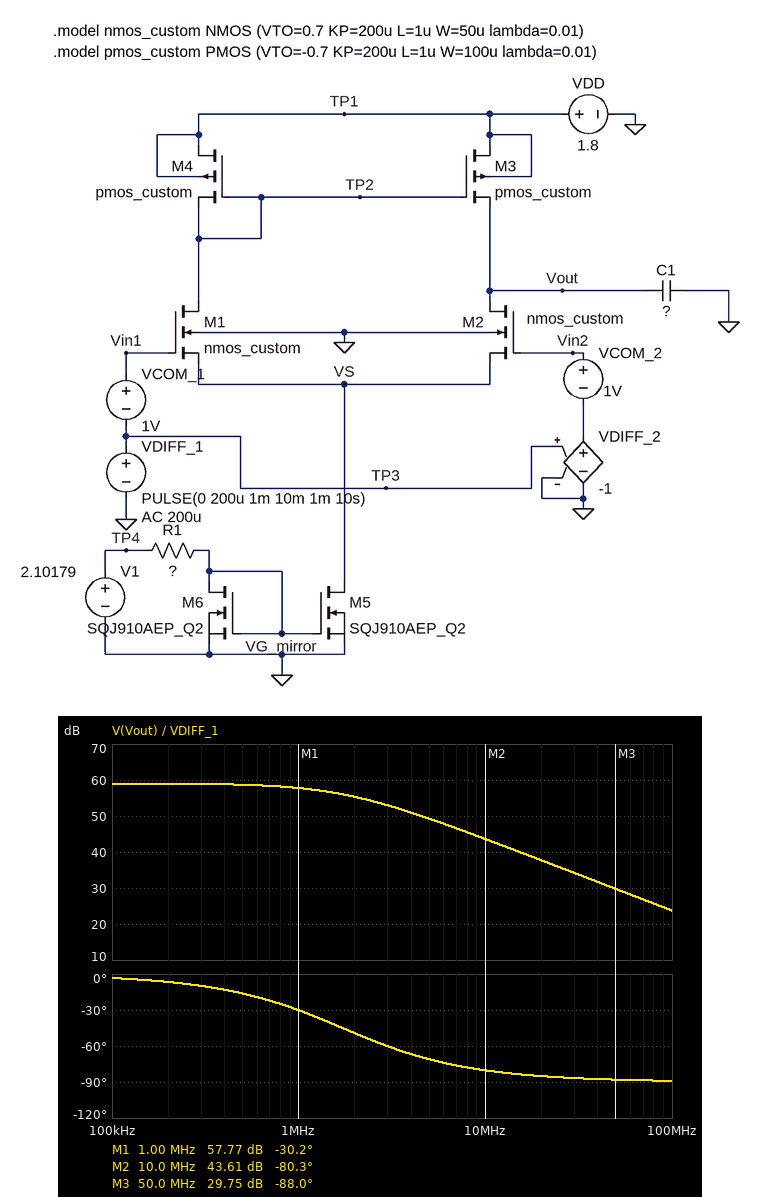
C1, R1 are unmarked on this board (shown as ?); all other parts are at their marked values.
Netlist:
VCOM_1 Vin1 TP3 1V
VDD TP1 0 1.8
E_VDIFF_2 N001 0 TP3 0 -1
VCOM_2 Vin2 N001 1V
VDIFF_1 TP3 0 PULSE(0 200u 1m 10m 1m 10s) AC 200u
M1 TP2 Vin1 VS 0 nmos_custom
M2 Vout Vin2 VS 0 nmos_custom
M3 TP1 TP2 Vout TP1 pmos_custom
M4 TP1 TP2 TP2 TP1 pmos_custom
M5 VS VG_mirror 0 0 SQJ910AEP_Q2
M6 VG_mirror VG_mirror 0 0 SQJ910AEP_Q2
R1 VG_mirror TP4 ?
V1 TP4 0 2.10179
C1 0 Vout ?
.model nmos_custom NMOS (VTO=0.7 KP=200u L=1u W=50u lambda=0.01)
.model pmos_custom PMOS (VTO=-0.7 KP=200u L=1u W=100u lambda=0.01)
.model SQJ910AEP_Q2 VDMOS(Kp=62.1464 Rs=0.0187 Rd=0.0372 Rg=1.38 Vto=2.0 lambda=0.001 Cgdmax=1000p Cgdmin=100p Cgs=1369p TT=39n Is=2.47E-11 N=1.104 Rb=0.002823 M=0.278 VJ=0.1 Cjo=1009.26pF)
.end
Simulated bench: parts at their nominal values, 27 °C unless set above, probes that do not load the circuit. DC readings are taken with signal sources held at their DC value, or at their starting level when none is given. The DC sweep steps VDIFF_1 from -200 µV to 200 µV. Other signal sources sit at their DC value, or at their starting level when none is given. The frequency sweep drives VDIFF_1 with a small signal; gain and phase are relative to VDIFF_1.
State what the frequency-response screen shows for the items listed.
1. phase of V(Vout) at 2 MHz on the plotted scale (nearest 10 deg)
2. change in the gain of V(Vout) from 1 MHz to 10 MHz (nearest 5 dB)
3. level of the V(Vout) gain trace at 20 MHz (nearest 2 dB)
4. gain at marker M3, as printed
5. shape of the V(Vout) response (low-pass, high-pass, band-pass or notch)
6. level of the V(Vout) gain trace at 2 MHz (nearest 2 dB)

-50 deg
-15 dB
38 dB
29.75 dB
low-pass
56 dB
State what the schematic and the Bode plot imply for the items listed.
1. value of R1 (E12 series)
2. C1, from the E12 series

820 Ω
470 fF
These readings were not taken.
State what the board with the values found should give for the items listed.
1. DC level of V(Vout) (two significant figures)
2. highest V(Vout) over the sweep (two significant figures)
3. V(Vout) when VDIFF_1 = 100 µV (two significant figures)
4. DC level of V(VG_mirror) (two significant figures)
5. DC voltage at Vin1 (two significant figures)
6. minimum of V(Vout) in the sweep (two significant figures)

940 mV
1.1 V
1.0 V
1.7 V
1.0 V
760 mV
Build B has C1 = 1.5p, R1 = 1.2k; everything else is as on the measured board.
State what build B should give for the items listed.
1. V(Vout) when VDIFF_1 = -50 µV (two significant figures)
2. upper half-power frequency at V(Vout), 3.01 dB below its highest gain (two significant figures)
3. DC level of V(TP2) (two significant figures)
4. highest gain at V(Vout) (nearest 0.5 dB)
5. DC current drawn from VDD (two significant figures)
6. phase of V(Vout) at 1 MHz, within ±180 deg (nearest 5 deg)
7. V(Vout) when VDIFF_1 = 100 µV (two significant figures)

910 mV
380 kHz
970 mV
60.5 dB
360 µA
-70 deg
1.1 V
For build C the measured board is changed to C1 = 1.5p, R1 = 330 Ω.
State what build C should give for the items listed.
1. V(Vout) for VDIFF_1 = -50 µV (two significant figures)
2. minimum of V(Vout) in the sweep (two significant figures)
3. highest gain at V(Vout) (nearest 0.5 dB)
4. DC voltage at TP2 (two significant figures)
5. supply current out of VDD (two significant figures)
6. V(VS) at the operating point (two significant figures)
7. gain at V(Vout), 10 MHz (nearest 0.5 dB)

860 mV
750 mV
56.5 dB
890 mV
890 µA
3.2 mV
36.0 dB
